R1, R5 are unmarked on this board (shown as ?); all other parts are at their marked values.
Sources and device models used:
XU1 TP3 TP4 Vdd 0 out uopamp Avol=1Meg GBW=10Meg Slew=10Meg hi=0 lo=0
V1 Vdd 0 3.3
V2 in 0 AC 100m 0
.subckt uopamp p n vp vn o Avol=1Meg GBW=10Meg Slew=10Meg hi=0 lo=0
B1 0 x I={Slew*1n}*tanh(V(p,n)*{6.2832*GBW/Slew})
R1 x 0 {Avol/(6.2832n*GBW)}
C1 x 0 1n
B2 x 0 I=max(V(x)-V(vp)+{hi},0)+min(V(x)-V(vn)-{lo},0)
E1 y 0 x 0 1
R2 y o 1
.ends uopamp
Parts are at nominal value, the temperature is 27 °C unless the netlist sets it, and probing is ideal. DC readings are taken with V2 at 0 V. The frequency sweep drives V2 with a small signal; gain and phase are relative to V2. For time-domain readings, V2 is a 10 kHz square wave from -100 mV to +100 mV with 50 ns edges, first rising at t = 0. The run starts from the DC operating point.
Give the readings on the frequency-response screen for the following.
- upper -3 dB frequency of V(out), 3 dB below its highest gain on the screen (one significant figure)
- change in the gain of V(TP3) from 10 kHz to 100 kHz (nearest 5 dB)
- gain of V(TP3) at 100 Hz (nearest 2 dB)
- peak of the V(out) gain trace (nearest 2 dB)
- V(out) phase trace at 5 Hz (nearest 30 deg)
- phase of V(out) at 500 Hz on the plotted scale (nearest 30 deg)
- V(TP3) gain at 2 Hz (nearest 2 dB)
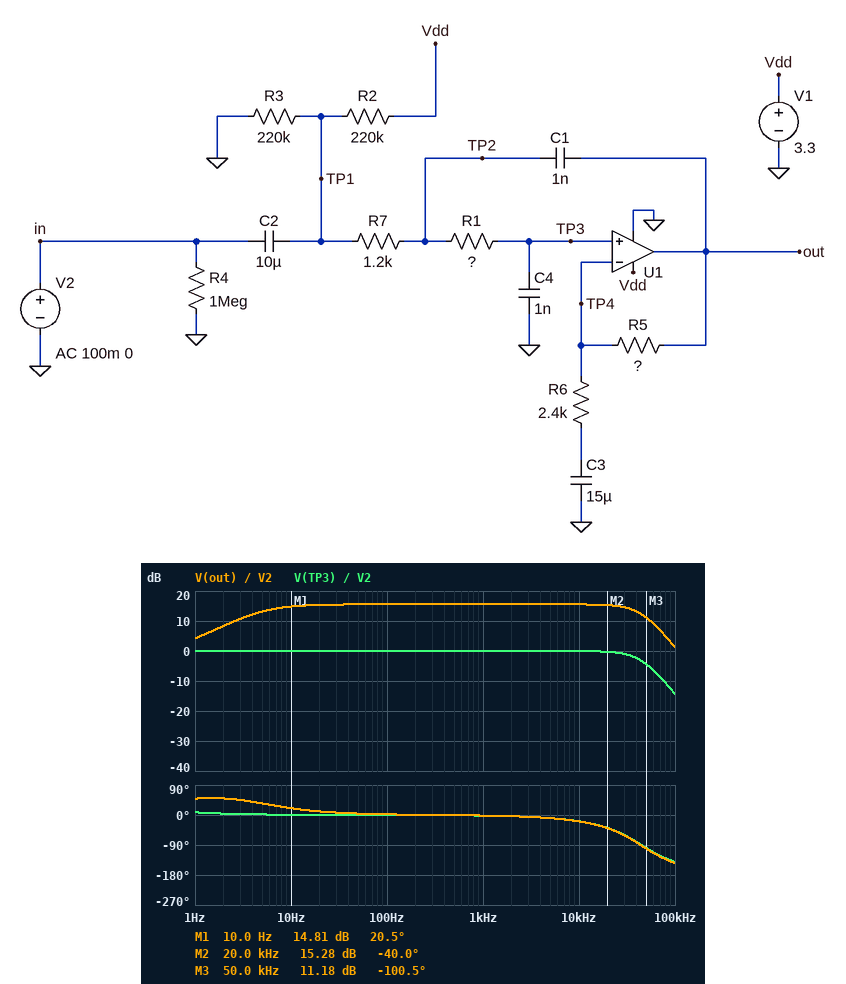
40 kHz
-15 dB
0 dB
16 dB
30 deg
0 deg
0 dB
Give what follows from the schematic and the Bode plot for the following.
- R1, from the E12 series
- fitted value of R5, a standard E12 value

10 kΩ
12 kΩ
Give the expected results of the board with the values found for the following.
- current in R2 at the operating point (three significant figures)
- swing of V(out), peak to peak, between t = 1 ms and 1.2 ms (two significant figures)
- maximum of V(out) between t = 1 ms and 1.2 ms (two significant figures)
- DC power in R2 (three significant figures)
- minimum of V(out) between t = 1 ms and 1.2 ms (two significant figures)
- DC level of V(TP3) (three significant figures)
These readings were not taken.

7.50 µA
1.3 V
2.9 V
12.4 µW
1.6 V
1.65 V
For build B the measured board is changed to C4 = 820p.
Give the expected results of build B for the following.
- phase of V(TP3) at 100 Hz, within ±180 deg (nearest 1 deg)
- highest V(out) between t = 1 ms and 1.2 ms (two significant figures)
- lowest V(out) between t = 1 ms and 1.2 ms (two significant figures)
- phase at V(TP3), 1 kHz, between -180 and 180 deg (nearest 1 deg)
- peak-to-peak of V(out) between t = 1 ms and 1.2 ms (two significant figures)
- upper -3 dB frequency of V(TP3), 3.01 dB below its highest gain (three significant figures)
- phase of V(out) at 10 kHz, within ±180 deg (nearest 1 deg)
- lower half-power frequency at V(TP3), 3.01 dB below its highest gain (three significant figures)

0 deg
3.0 V
1.4 V
-1 deg
1.6 V
57.4 kHz
-12 deg
212 mHz
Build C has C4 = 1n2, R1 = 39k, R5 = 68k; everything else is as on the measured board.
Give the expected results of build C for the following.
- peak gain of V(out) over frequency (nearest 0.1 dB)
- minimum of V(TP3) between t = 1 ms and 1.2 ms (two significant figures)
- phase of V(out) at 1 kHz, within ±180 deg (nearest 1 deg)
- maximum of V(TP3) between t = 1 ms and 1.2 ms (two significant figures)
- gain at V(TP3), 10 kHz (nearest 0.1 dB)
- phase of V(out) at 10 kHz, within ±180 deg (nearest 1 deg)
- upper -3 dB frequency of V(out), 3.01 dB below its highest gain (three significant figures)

29.4 dB
1.7 V
-5 deg
1.8 V
-1.2 dB
-53 deg
15.2 kHz
